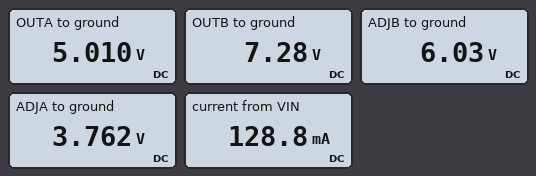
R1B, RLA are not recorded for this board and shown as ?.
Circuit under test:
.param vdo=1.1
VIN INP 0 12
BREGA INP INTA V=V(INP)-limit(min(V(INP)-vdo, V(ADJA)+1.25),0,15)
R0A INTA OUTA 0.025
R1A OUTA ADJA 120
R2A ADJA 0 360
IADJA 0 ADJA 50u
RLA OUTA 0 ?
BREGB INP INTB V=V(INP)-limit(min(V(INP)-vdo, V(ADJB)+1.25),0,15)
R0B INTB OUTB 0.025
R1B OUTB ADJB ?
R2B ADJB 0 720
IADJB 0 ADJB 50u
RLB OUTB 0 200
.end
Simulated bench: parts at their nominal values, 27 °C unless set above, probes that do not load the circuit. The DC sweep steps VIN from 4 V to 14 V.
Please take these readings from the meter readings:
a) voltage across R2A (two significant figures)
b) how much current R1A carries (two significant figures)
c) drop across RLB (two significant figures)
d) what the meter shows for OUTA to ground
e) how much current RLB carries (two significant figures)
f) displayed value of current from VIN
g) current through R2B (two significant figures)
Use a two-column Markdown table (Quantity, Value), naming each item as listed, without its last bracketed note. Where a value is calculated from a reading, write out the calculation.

| Quantity | Value |
|---|---|
| voltage across R2A | 3.762 V = 3.8 V |
| how much current R1A carries | (5.01 V - 3.762 V) / 120 Ω = 10 mA |
| drop across RLB | 7.28 V = 7.3 V |
| what the meter shows for OUTA to ground | 5.010 V |
| how much current RLB carries | (7.28 V) / 200 Ω = 36 mA |
| displayed value of current from VIN | 128.8 mA |
| current through R2B | (6.03 V) / 720 Ω = 8.4 mA |
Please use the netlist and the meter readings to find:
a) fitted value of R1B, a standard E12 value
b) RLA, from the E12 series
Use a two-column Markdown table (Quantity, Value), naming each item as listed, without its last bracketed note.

| Quantity | Value |
|---|---|
| fitted value of R1B, a standard E12 value | 150 Ω |
| RLA, from the E12 series | 68 Ω |
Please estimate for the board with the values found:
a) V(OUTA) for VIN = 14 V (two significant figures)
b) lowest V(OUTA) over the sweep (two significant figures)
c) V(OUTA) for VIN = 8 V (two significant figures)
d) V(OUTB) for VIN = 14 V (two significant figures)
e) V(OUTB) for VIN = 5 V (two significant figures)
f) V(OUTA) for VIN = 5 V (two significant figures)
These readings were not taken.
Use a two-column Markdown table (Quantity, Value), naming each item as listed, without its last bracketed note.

| Quantity | Value |
|---|---|
| V(OUTA) for VIN = 14 V | 5.0 V |
| lowest V(OUTA) over the sweep | 2.9 V |
| V(OUTA) for VIN = 8 V | 5.0 V |
| V(OUTB) for VIN = 14 V | 7.3 V |
| V(OUTB) for VIN = 5 V | 3.9 V |
| V(OUTA) for VIN = 5 V | 3.9 V |
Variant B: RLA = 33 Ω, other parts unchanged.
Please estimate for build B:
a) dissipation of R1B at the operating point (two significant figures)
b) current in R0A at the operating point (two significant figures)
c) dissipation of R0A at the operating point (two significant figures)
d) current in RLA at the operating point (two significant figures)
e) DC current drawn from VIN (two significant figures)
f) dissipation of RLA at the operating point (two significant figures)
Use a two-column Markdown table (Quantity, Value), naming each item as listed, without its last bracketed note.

| Quantity | Value |
|---|---|
| dissipation of R1B at the operating point | 10 mW |
| current in R0A at the operating point | 160 mA |
| dissipation of R0A at the operating point | 660 µW |
| current in RLA at the operating point | 150 mA |
| DC current drawn from VIN | 210 mA |
| dissipation of RLA at the operating point | 760 mW |
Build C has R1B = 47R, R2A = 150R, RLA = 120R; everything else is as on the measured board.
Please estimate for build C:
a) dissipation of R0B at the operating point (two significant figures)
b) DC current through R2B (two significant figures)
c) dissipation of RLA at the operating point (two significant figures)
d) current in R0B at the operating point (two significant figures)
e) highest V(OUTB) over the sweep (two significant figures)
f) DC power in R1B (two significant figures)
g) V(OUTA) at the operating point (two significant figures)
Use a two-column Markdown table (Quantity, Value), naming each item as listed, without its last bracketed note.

| Quantity | Value |
|---|---|
| dissipation of R0B at the operating point | 120 µW |
| DC current through R2B | 14 mA |
| dissipation of RLA at the operating point | 66 mW |
| current in R0B at the operating point | 69 mA |
| highest V(OUTB) over the sweep | 13 V |
| DC power in R1B | 9.4 mW |
| V(OUTA) at the operating point | 2.8 V |
